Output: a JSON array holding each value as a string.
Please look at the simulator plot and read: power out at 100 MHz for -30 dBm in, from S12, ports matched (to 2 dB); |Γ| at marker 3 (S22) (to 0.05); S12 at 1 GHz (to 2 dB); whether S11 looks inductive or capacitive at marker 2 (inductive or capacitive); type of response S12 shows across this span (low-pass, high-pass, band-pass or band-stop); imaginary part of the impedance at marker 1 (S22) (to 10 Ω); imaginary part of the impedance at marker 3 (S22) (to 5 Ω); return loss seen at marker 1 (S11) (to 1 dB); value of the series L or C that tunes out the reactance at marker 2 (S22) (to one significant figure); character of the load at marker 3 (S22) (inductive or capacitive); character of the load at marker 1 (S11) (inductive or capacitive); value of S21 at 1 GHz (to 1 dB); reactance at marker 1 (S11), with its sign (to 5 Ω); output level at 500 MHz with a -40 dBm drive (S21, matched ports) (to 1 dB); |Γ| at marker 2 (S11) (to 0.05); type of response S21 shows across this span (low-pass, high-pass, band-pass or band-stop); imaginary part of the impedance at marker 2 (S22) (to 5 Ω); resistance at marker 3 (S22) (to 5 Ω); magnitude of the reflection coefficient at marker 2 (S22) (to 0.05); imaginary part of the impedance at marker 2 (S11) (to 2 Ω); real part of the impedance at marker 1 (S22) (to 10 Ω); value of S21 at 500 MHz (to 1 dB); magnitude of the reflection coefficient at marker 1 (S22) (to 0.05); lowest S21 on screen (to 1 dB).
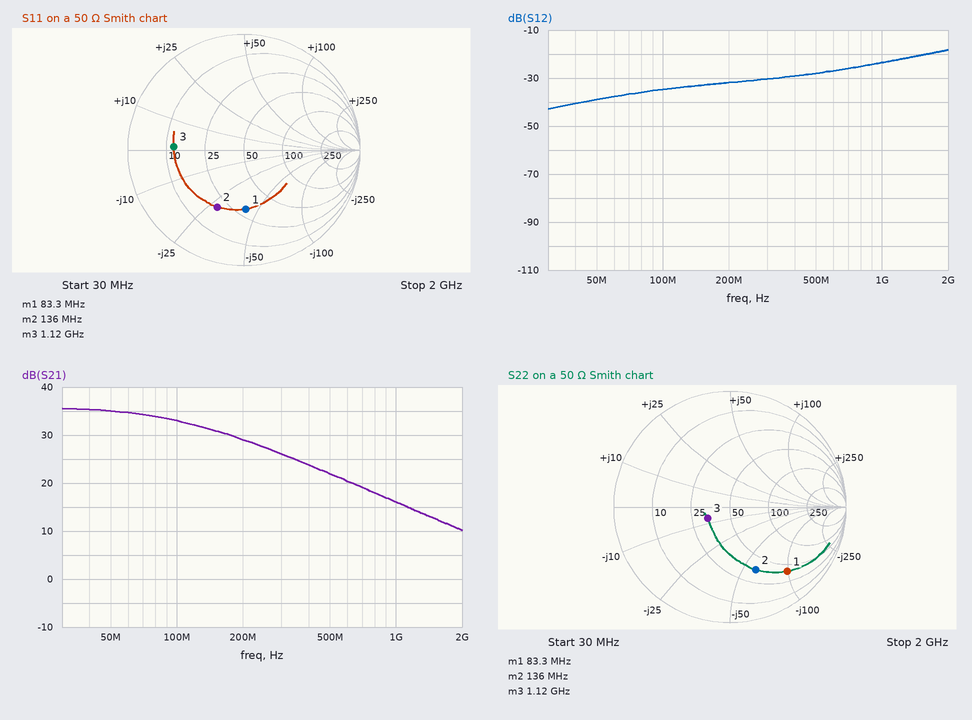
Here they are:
["-64 dBm", "0.20", "-24 dB", "capacitive", "high-pass", "-100 Ω", "-5 Ω", "6 dB", "70 nH", "capacitive", "capacitive", "16 dB", "-40 Ω", "-18 dBm", "0.55", "low-pass", "-60 Ω", "35 Ω", "0.60", "-28 Ω", "40 Ω", "22 dB", "0.75", "10 dB"]
